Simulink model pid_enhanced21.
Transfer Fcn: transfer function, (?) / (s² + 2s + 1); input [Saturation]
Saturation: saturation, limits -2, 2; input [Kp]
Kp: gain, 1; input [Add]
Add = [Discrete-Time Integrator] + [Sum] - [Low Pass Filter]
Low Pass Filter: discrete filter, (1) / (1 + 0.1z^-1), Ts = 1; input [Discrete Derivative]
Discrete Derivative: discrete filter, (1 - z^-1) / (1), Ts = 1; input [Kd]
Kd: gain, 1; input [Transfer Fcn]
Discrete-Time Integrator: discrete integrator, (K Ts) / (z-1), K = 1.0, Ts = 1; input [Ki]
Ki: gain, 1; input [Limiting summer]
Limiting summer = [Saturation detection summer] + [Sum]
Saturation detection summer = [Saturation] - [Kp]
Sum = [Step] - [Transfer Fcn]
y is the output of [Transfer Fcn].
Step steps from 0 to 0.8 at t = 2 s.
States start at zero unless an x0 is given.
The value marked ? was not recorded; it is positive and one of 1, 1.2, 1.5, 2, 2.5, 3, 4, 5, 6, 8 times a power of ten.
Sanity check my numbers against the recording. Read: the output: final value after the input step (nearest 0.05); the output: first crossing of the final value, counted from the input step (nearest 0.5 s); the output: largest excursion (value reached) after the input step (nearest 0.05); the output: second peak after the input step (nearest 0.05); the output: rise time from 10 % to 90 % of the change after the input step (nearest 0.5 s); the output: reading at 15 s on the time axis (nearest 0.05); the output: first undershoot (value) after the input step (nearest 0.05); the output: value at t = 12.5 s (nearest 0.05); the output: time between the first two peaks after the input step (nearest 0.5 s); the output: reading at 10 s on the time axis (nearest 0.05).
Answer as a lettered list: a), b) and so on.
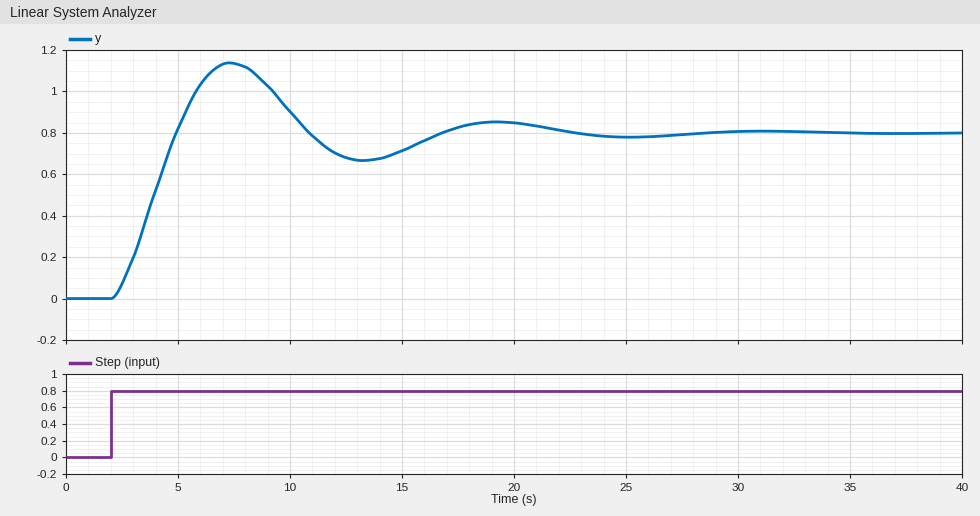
a) 0.80
b) 3.0 s
c) 1.15
d) 0.85
e) 2.0 s
f) 0.70
g) 0.65
h) 0.70
i) 12.0 s
j) 0.90
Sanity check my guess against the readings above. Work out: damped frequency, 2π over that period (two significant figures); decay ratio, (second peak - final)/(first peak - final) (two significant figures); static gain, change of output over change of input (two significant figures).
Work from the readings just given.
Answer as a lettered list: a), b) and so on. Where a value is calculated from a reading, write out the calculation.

a) 2π / 12 = 0.52 rad/s
b) (0.85 - 0.8) / (1.15 - 0.8) = 0.14
c) (0.8 - 0) / (0.8 - 0) = 1.0
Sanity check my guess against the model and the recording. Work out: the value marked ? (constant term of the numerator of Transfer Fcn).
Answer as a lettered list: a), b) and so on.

a) 1
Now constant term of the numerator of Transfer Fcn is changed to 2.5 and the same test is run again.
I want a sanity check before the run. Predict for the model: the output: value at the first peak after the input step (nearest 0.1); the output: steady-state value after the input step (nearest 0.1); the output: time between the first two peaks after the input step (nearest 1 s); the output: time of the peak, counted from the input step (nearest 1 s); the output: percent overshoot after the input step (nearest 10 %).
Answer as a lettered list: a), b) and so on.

a) 1.2
b) 0.8
c) 9 s
d) 4 s
e) 50 %
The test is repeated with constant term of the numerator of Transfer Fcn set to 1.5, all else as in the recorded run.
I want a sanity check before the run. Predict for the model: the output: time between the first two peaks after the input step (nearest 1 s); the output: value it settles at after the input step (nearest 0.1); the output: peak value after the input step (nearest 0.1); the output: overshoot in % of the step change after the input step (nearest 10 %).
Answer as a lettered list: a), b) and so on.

a) 11 s
b) 0.8
c) 1.2
d) 50 %
